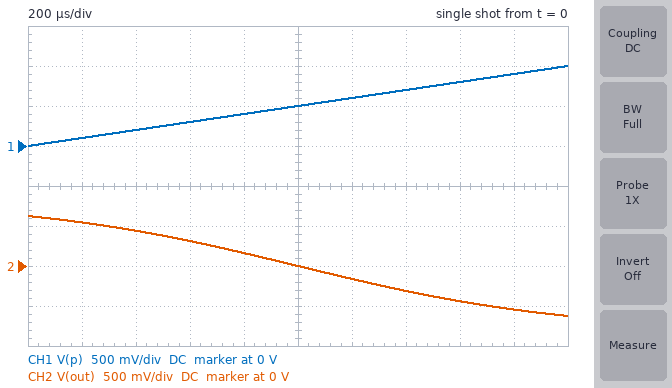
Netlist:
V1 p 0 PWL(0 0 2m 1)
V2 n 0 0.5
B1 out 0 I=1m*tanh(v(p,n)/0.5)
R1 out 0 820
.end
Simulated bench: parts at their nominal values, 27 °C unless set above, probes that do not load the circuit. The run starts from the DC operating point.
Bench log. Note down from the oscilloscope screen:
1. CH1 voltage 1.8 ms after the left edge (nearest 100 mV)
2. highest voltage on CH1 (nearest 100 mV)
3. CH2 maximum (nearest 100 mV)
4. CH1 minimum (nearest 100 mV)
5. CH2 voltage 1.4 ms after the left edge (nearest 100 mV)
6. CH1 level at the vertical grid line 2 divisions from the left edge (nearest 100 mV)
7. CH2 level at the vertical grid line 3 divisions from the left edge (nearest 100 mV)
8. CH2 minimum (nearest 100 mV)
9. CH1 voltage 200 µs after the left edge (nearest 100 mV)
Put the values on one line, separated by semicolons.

900 mV; 1.0 V; 600 mV; 0 V; -300 mV; 200 mV; 300 mV; -600 mV; 100 mV
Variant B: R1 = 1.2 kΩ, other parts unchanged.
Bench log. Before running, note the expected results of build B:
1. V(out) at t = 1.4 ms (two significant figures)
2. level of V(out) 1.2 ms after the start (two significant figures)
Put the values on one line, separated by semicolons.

-460 mV; -240 mV
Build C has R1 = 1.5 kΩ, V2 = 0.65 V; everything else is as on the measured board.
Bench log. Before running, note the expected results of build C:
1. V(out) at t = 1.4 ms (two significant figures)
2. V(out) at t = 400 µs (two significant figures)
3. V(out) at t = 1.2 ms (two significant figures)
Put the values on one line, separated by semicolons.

-150 mV; 1.1 V; 150 mV
